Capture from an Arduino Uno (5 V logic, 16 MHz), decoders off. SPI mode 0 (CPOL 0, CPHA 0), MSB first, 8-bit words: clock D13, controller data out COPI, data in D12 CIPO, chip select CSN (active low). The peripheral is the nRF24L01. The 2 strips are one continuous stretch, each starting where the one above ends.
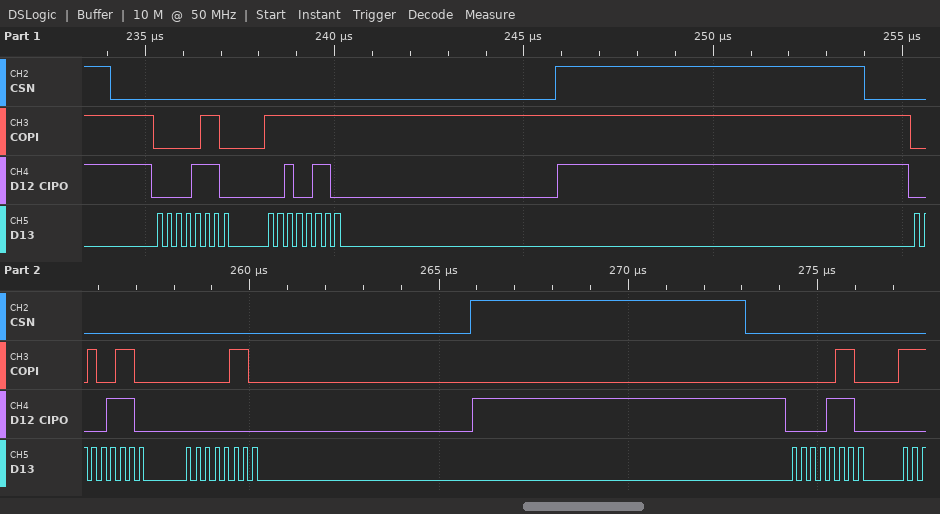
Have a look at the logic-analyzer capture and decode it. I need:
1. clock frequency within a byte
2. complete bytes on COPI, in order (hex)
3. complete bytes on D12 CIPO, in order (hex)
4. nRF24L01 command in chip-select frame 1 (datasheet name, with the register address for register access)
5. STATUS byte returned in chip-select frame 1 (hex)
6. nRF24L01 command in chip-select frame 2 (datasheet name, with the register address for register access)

4 MHz
06 FF 26 06 06
0E 26 0E 00 0E
R_REGISTER 0x06
0x0E
W_REGISTER 0x06
